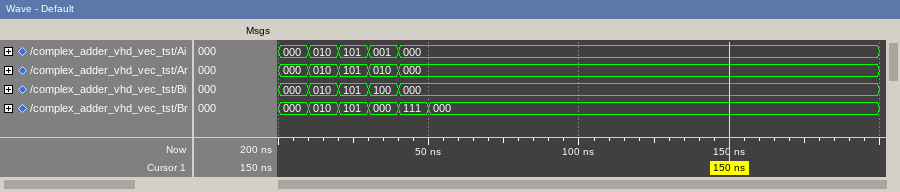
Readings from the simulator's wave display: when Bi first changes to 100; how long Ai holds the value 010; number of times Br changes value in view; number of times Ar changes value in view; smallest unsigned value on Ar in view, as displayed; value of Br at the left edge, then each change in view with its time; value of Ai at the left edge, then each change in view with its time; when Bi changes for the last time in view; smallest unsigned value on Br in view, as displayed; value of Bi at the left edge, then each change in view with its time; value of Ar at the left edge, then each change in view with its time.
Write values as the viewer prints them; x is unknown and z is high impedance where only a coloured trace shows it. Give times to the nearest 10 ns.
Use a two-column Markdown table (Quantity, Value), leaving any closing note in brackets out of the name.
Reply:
| Quantity | Value |
|---|---|
| when Bi first changes to 100 | 30 ns |
| how long Ai holds the value 010 | 10 ns |
| number of times Br changes value in view | 5 |
| number of times Ar changes value in view | 4 |
| smallest unsigned value on Ar in view, as displayed | 000 |
| value of Br at the left edge, then each change in view with its time | 000, 010 at 10 ns, 101 at 20 ns, 000 at 30 ns, 111 at 40 ns, 000 at 50 ns |
| value of Ai at the left edge, then each change in view with its time | 000, 010 at 10 ns, 101 at 20 ns, 001 at 30 ns, 000 at 40 ns |
| when Bi changes for the last time in view | 40 ns |
| smallest unsigned value on Br in view, as displayed | 000 |
| value of Bi at the left edge, then each change in view with its time | 000, 010 at 10 ns, 101 at 20 ns, 100 at 30 ns, 000 at 40 ns |
| value of Ar at the left edge, then each change in view with its time | 000, 010 at 10 ns, 101 at 20 ns, 010 at 30 ns, 000 at 40 ns |
